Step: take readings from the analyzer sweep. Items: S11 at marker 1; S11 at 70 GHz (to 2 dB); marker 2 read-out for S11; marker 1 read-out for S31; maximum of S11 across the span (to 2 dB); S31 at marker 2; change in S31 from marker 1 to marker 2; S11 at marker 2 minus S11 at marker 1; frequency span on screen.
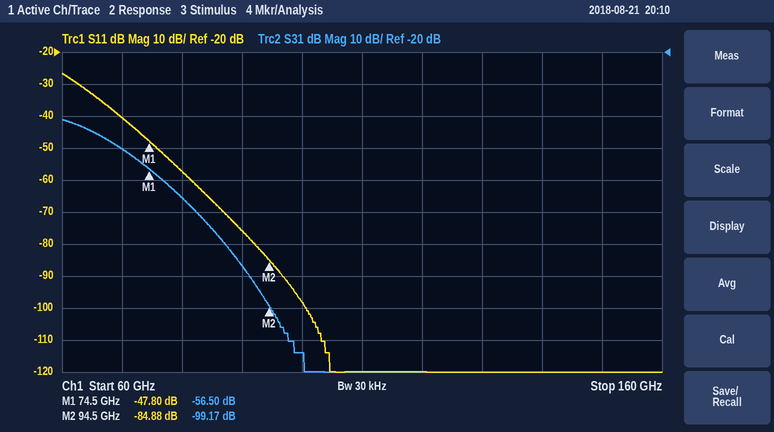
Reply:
-47.80 dB
-40 dB
-84.88 dB
-56.50 dB
-26 dB
-99.17 dB
-42.67 dB
-37.08 dB
100 GHz
